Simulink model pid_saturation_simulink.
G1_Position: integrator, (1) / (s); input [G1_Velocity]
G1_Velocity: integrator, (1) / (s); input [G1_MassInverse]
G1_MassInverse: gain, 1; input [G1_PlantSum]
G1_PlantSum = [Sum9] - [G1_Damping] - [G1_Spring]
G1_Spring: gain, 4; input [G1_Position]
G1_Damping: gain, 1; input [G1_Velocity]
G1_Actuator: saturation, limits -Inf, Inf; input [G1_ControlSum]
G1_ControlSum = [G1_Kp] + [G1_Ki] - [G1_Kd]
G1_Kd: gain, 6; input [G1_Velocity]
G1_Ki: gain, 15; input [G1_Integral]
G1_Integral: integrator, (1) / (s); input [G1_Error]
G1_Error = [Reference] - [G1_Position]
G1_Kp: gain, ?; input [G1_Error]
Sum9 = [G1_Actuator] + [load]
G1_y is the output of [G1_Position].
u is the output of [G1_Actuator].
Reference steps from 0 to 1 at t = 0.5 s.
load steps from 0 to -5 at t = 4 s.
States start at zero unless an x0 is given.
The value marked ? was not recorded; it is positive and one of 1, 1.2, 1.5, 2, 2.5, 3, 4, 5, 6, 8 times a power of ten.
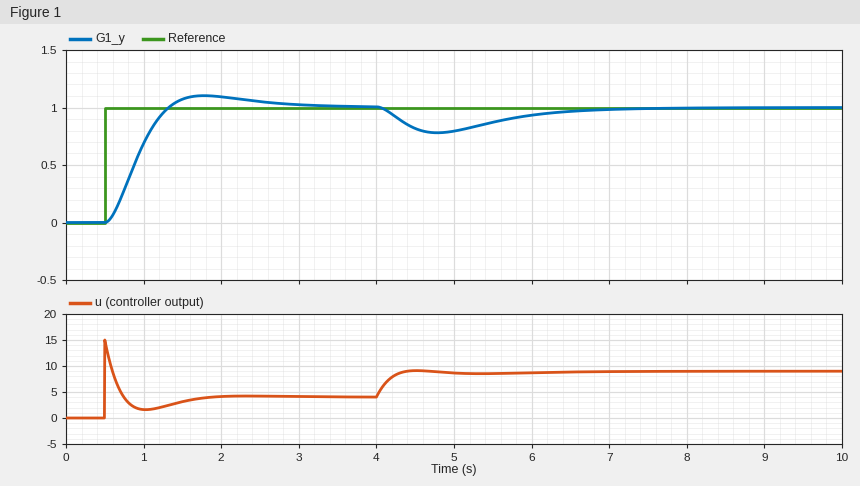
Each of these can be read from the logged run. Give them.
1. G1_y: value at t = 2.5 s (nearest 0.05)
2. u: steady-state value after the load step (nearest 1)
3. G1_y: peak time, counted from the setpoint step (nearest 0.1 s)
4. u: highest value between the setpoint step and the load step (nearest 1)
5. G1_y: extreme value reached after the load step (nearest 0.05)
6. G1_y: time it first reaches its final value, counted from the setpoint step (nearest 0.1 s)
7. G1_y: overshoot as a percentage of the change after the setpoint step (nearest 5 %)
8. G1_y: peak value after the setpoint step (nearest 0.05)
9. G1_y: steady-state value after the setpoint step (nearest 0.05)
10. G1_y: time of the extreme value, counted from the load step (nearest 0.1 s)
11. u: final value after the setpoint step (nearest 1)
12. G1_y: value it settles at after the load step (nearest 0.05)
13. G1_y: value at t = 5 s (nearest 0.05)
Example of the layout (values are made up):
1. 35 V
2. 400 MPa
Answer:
1. 1.05
2. 9
3. 1.3 s
4. 15
5. 0.80
6. 0.8 s
7. 10 %
8. 1.10
9. 1.00
10. 0.8 s
11. 4
12. 1.00
13. 0.80
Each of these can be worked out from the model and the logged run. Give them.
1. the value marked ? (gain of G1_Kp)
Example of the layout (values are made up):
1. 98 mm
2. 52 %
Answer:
1. 15
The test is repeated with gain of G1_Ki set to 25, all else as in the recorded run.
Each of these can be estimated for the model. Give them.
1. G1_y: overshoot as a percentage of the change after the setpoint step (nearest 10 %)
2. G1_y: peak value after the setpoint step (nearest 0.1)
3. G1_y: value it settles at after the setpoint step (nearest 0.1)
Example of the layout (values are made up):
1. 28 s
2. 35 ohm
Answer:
1. 20 %
2. 1.2
3. 1.0
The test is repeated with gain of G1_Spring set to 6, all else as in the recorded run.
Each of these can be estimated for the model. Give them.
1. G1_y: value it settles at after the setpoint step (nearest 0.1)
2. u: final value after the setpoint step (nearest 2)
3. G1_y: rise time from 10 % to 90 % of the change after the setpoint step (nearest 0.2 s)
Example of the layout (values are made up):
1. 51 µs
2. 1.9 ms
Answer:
1. 1.0
2. 6
3. 0.6 s
